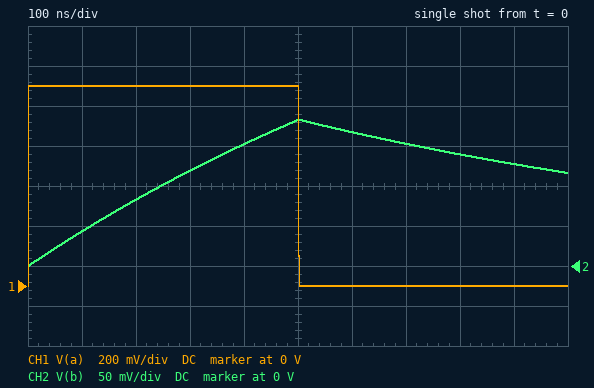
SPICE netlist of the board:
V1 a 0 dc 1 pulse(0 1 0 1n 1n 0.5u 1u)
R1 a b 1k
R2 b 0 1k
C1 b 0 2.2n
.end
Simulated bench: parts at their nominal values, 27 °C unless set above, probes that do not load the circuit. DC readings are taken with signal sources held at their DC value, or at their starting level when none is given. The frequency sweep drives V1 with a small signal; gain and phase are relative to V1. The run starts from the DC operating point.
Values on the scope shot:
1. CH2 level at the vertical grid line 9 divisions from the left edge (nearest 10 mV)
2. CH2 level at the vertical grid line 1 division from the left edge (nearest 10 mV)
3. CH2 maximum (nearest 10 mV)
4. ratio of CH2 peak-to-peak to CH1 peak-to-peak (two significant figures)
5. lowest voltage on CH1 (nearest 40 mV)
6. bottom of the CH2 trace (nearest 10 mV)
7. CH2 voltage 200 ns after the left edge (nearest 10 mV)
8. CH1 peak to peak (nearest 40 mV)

130 mV
40 mV
180 mV
0.18
0 V
0 V
80 mV
1.00 V
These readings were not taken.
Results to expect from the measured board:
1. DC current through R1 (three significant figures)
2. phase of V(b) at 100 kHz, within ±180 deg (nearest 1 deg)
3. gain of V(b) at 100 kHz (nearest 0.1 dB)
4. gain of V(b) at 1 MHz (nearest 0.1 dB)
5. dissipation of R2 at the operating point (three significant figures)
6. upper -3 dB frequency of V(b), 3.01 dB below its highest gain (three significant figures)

500 µA
-35 deg
-7.7 dB
-22.9 dB
250 µW
145 kHz
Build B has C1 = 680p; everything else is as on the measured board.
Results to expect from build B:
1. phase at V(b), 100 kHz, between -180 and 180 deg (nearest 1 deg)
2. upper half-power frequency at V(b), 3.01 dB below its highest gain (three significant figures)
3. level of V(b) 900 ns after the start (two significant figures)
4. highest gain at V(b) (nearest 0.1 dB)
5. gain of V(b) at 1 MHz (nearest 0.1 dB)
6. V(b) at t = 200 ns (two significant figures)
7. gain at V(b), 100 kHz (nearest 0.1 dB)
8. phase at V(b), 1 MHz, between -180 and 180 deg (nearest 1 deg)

-12 deg
468 kHz
120 mV
-6.0 dB
-13.5 dB
220 mV
-6.2 dB
-65 deg
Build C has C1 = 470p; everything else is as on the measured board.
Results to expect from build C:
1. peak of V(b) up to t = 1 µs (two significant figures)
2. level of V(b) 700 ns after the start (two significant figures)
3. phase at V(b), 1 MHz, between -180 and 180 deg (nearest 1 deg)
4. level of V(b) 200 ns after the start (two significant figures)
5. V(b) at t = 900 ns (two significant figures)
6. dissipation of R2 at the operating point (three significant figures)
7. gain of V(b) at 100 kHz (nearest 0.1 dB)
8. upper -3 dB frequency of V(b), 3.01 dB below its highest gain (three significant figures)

440 mV
190 mV
-56 deg
290 mV
81 mV
250 µW
-6.1 dB
677 kHz
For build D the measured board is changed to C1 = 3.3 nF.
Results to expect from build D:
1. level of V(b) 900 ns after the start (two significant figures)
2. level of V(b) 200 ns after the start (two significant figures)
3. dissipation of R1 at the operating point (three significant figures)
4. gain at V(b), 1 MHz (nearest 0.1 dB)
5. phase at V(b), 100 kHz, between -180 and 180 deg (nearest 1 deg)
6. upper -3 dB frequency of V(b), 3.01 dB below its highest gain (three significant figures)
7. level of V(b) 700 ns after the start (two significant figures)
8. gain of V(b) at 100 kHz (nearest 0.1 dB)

100 mV
57 mV
250 µW
-26.4 dB
-46 deg
96.5 kHz
120 mV
-9.2 dB
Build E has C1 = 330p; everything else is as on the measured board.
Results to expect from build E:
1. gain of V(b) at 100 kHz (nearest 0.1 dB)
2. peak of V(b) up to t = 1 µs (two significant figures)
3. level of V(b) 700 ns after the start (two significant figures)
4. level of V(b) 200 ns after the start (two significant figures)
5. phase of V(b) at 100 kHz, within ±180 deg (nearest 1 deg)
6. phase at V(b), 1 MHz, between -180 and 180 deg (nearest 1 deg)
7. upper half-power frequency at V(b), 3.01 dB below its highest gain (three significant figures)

-6.1 dB
480 mV
140 mV
350 mV
-6 deg
-46 deg
965 kHz
